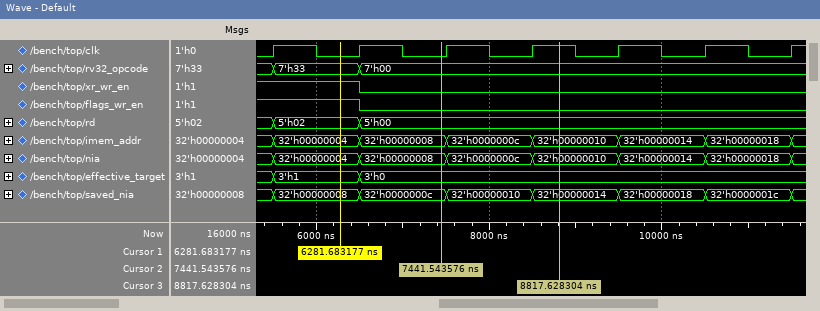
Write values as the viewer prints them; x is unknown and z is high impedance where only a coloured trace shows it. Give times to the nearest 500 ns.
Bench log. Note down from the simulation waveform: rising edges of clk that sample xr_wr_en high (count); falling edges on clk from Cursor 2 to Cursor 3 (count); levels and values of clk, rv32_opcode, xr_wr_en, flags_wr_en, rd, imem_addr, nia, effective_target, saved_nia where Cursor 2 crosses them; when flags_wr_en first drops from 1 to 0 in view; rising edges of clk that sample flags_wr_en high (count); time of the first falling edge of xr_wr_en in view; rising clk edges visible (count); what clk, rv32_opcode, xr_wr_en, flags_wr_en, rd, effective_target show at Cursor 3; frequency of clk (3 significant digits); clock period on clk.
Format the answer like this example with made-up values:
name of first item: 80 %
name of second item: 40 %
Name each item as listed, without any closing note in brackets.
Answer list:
rising edges of clk that sample xr_wr_en high: 2
falling edges on clk from Cursor 2 to Cursor 3: 1
levels and values of clk, rv32_opcode, xr_wr_en, flags_wr_en, rd, imem_addr, nia, effective_target, saved_nia where Cursor 2 crosses them: clk=0, rv32_opcode=7'h00, xr_wr_en=0, flags_wr_en=0, rd=5'h00, imem_addr=32'h00000008, nia=32'h00000008, effective_target=3'h0, saved_nia=32'h0000000c
when flags_wr_en first drops from 1 to 0 in view: 6500 ns
rising edges of clk that sample flags_wr_en high: 2
time of the first falling edge of xr_wr_en in view: 6500 ns
rising clk edges visible: 7
what clk, rv32_opcode, xr_wr_en, flags_wr_en, rd, effective_target show at Cursor 3: clk=1, rv32_opcode=7'h00, xr_wr_en=0, flags_wr_en=0, rd=5'h00, effective_target=3'h0
frequency of clk: 1.00 MHz
clock period on clk: 1000 ns
